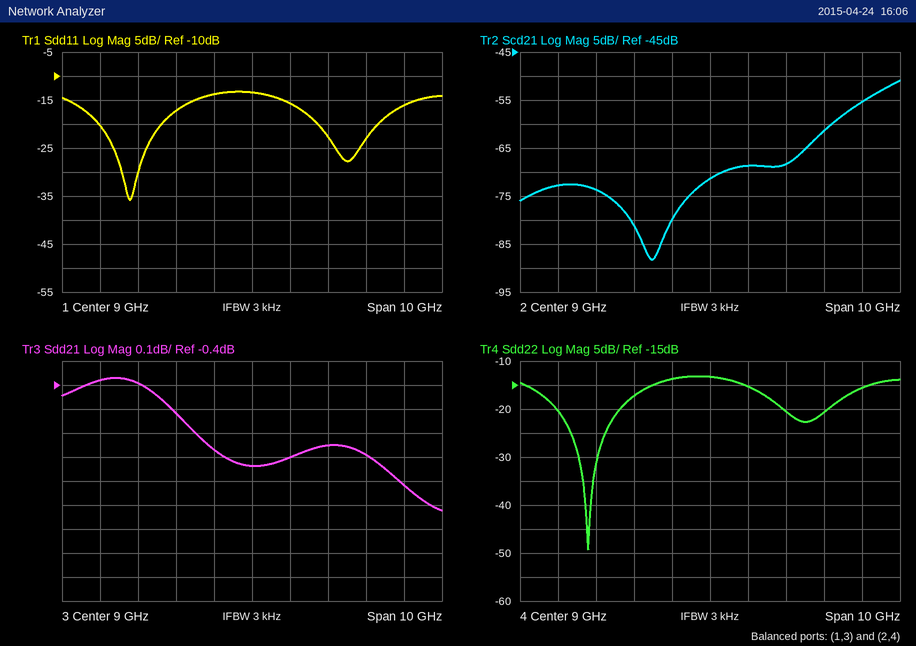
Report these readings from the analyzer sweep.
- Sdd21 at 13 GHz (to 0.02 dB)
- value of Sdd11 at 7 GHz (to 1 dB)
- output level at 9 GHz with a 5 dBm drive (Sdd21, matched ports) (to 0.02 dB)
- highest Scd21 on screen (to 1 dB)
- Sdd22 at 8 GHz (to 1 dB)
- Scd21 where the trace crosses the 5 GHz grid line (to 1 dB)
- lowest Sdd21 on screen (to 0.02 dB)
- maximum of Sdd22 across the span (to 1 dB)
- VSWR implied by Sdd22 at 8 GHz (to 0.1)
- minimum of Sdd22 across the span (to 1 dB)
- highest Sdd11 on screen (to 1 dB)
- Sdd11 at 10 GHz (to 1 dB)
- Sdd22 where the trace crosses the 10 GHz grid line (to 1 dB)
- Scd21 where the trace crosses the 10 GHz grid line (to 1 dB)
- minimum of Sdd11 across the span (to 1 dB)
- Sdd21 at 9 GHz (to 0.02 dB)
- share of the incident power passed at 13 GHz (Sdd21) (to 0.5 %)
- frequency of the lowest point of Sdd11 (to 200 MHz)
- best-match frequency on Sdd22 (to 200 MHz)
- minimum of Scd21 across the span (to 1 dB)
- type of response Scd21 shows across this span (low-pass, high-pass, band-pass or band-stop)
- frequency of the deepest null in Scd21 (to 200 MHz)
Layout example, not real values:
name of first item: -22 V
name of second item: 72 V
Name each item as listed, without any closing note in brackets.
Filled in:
Sdd21 at 13 GHz: -0.82 dB
value of Sdd11 at 7 GHz: -17 dB
output level at 9 GHz with a 5 dBm drive (Sdd21, matched ports): 4.26 dBm
highest Scd21 on screen: -51 dB
Sdd22 at 8 GHz: -14 dB
Scd21 where the trace crosses the 5 GHz grid line: -73 dB
lowest Sdd21 on screen: -0.92 dB
maximum of Sdd22 across the span: -13 dB
VSWR implied by Sdd22 at 8 GHz: 1.5
minimum of Sdd22 across the span: -49 dB
highest Sdd11 on screen: -13 dB
Sdd11 at 10 GHz: -16 dB
Sdd22 where the trace crosses the 10 GHz grid line: -15 dB
Scd21 where the trace crosses the 10 GHz grid line: -69 dB
minimum of Sdd11 across the span: -36 dB
Sdd21 at 9 GHz: -0.74 dB
share of the incident power passed at 13 GHz (Sdd21): 83.0 %
frequency of the lowest point of Sdd11: 5.8 GHz
best-match frequency on Sdd22: 5.8 GHz
minimum of Scd21 across the span: -88 dB
type of response Scd21 shows across this span: high-pass
frequency of the deepest null in Scd21: 7.4 GHz
